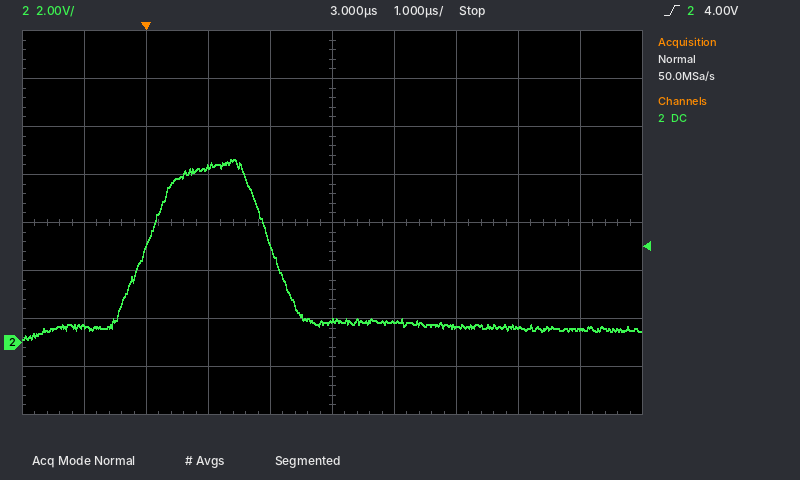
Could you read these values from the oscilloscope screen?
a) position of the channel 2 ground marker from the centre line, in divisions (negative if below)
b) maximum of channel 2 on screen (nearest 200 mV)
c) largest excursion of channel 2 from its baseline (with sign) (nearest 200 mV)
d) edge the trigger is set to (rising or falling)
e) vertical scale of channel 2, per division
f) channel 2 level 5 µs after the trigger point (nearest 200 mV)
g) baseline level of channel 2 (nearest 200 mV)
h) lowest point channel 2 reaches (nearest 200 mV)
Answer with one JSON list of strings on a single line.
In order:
["-2.5 div", "7.6 V", "+7.0 V", "rising", "2 V", "600 mV", "600 mV", "200 mV"]
